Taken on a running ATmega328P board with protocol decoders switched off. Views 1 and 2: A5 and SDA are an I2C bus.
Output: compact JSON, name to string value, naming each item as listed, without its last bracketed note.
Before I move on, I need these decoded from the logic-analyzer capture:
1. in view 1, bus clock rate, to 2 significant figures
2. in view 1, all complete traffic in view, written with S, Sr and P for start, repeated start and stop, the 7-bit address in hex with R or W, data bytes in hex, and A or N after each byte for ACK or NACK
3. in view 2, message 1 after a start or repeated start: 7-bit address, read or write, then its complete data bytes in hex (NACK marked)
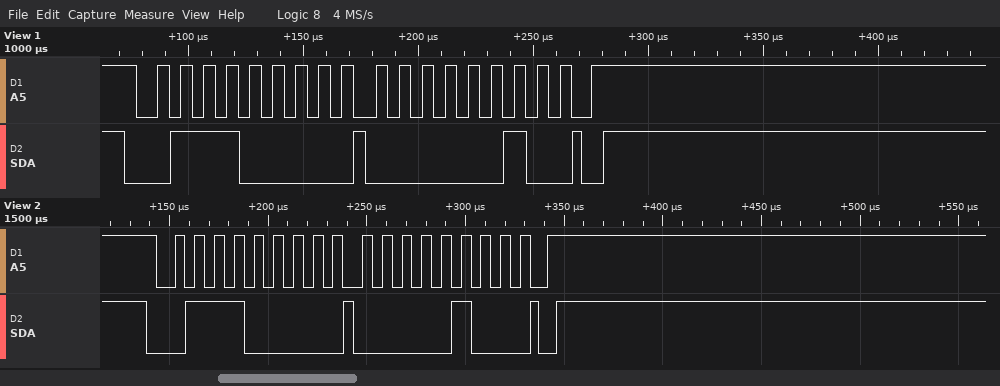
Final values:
{"in view 1, bus clock rate, to 2 significant figures": "100 kHz", "in view 1, all complete traffic in view, written with S, Sr and P for start, repeated start and stop, the 7-bit address in hex with R or W, data bytes in hex, and A or N after each byte for ACK or NACK": "S 38W A 02 A P", "in view 2, message 1 after a start or repeated start: 7-bit address, read or write, then its complete data bytes in hex": "0x38 write: 04"}
